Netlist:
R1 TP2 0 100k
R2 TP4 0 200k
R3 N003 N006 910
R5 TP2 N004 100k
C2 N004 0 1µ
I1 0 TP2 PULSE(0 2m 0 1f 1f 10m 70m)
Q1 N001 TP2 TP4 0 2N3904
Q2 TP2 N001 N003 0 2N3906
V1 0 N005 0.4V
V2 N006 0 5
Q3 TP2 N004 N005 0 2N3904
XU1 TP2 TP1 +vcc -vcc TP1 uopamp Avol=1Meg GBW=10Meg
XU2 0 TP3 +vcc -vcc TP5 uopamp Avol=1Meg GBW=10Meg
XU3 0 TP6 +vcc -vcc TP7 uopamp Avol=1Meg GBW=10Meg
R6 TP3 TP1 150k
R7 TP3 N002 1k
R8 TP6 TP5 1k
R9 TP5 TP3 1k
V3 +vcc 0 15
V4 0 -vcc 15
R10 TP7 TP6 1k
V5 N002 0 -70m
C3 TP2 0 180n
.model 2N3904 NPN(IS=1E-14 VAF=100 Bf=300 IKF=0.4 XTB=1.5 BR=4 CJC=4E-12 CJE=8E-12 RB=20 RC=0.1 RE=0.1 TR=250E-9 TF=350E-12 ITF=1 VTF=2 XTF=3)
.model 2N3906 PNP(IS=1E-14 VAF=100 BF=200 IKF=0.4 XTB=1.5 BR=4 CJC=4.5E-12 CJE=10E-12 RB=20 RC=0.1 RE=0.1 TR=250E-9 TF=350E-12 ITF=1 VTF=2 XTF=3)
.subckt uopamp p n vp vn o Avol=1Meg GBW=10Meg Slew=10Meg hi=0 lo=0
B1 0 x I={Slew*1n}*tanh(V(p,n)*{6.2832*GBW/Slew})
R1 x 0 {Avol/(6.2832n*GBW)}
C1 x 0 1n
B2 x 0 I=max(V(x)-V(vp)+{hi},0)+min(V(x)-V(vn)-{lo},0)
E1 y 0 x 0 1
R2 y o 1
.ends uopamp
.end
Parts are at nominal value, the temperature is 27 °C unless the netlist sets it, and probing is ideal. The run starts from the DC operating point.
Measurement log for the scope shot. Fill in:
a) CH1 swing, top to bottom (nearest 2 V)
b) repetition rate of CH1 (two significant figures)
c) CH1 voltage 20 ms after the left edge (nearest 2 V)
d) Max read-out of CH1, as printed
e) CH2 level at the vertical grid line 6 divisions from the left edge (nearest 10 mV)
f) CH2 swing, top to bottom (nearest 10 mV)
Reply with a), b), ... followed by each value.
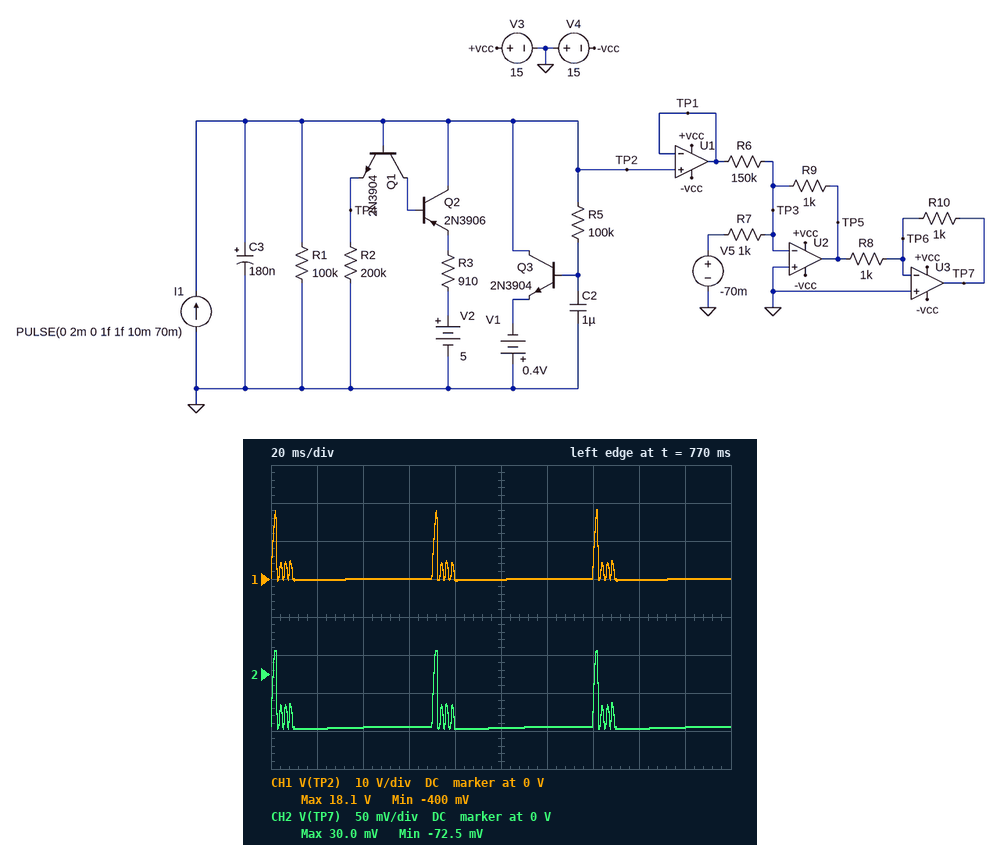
a) 18 V
b) 14 Hz
c) 0 V
d) 18.1 V
e) -70 mV
f) 100 mV
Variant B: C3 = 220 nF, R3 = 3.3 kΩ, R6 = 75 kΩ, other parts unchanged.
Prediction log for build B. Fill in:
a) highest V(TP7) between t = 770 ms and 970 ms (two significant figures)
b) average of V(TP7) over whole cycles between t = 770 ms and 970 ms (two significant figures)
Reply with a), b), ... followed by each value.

a) 130 mV
b) -64 mV
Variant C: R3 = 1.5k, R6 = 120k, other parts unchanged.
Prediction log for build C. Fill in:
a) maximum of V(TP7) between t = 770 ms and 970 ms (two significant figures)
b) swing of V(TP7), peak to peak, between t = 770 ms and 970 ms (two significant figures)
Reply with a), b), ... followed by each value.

a) 55 mV
b) 130 mV
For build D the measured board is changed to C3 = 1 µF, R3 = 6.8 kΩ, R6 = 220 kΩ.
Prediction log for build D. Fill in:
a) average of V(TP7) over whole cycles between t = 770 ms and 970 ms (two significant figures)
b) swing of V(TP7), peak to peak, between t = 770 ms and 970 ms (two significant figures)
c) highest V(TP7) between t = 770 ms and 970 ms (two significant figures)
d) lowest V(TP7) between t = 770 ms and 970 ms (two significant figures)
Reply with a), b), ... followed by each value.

a) -68 mV
b) 46 mV
c) -26 mV
d) -72 mV
